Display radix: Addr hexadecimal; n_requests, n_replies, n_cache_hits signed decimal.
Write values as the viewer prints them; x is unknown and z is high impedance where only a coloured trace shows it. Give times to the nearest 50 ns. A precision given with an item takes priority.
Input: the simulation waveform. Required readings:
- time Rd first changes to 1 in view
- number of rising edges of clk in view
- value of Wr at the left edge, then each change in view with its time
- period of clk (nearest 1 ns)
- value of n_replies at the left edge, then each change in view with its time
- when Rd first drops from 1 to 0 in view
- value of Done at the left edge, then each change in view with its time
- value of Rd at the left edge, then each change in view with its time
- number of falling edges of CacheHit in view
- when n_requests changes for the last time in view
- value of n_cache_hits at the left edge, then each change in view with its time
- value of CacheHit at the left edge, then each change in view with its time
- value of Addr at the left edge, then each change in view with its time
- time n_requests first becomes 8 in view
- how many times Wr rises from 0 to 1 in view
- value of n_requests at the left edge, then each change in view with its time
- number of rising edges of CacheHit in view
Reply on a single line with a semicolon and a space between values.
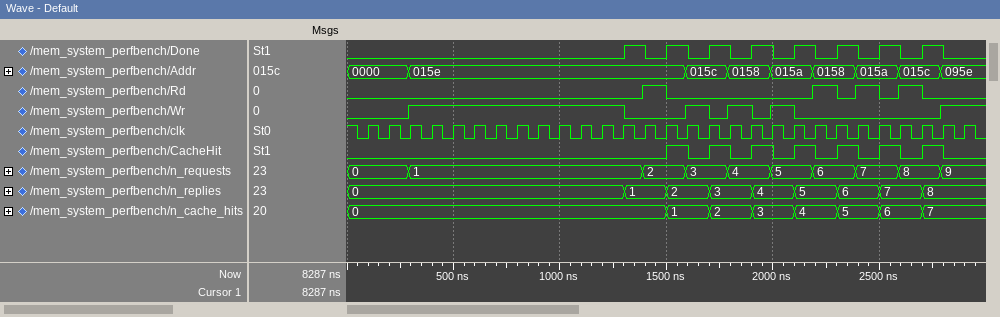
1400 ns; 29; 0, 1 at 300 ns, 0 at 1300 ns, 1 at 1600 ns, 0 at 1700 ns, 1 at 1800 ns, 0 at 1900 ns, 1 at 2000 ns, 0 at 2100 ns, 1 at 2800 ns; 100 ns; 0, 1 at 1300 ns, 2 at 1500 ns, 3 at 1700 ns, 4 at 1900 ns, 5 at 2100 ns, 6 at 2300 ns, 7 at 2500 ns, 8 at 2700 ns; 1500 ns; 0, 1 at 1300 ns, 0 at 1400 ns, 1 at 1500 ns, 0 at 1600 ns, 1 at 1700 ns, 0 at 1800 ns, 1 at 1900 ns, 0 at 2000 ns, 1 at 2100 ns, 0 at 2200 ns, 1 at 2300 ns, 0 at 2400 ns, 1 at 2500 ns, 0 at 2600 ns, 1 at 2700 ns, 0 at 2800 ns; 0, 1 at 1400 ns, 0 at 1500 ns, 1 at 2200 ns, 0 at 2300 ns, 1 at 2400 ns, 0 at 2500 ns, 1 at 2600 ns, 0 at 2700 ns; 7; 2800 ns; 0, 1 at 1500 ns, 2 at 1700 ns, 3 at 1900 ns, 4 at 2100 ns, 5 at 2300 ns, 6 at 2500 ns, 7 at 2700 ns; 0, 1 at 1500 ns, 0 at 1600 ns, 1 at 1700 ns, 0 at 1800 ns, 1 at 1900 ns, 0 at 2000 ns, 1 at 2100 ns, 0 at 2200 ns, 1 at 2300 ns, 0 at 2400 ns, 1 at 2500 ns, 0 at 2600 ns, 1 at 2700 ns, 0 at 2800 ns; 0000, 015e at 300 ns, 015c at 1600 ns, 0158 at 1800 ns, 015a at 2000 ns, 0158 at 2200 ns, 015a at 2400 ns, 015c at 2600 ns, 095e at 2800 ns; 2600 ns; 5; 0, 1 at 300 ns, 2 at 1400 ns, 3 at 1600 ns, 4 at 1800 ns, 5 at 2000 ns, 6 at 2200 ns, 7 at 2400 ns, 8 at 2600 ns, 9 at 2800 ns; 7
